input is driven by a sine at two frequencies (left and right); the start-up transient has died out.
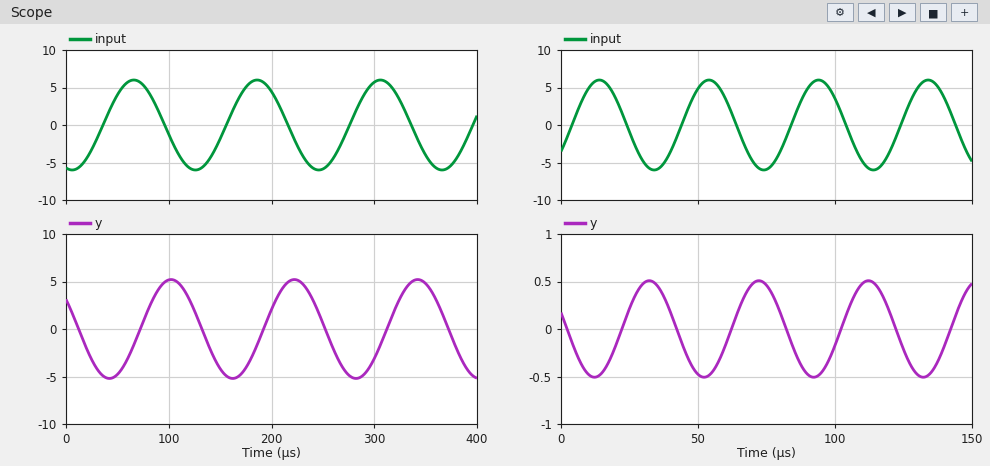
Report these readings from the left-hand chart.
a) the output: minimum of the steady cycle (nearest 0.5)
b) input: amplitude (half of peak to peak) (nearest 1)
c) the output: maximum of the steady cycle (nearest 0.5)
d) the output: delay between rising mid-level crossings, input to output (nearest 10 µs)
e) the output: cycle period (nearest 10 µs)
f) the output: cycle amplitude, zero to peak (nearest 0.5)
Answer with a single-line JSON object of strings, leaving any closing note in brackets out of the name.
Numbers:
{"the output: minimum of the steady cycle": "-5.0", "input: amplitude (half of peak to peak)": "6", "the output: maximum of the steady cycle": "5.0", "the output: delay between rising mid-level crossings, input to output": "40 µs", "the output: cycle period": "120 µs", "the output: cycle amplitude, zero to peak": "5.0"}
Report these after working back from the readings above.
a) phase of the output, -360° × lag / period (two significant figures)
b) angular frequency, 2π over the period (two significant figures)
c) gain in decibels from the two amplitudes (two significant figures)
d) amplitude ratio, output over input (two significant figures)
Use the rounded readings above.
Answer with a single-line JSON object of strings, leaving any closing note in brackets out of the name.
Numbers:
{"phase of the output, -360° × lag / period": "-120°", "angular frequency, 2π over the period": "0.052 rad/µs", "gain in decibels from the two amplitudes": "-1.6 dB", "amplitude ratio, output over input": "0.83"}
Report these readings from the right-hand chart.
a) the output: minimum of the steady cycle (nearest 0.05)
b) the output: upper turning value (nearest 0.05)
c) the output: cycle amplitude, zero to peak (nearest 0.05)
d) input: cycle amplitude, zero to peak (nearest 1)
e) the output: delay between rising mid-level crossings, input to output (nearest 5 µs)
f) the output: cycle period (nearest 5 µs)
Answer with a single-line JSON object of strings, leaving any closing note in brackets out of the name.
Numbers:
{"the output: minimum of the steady cycle": "-0.50", "the output: upper turning value": "0.50", "the output: cycle amplitude, zero to peak": "0.50", "input: cycle amplitude, zero to peak": "6", "the output: delay between rising mid-level crossings, input to output": "20 µs", "the output: cycle period": "40 µs"}
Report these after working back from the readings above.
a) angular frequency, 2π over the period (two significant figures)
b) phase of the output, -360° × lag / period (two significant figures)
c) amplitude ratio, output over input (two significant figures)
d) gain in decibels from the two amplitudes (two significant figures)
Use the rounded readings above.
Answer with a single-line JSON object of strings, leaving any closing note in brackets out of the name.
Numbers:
{"angular frequency, 2π over the period": "0.16 rad/µs", "phase of the output, -360° × lag / period": "-180°", "amplitude ratio, output over input": "0.083", "gain in decibels from the two amplitudes": "-22 dB"}
